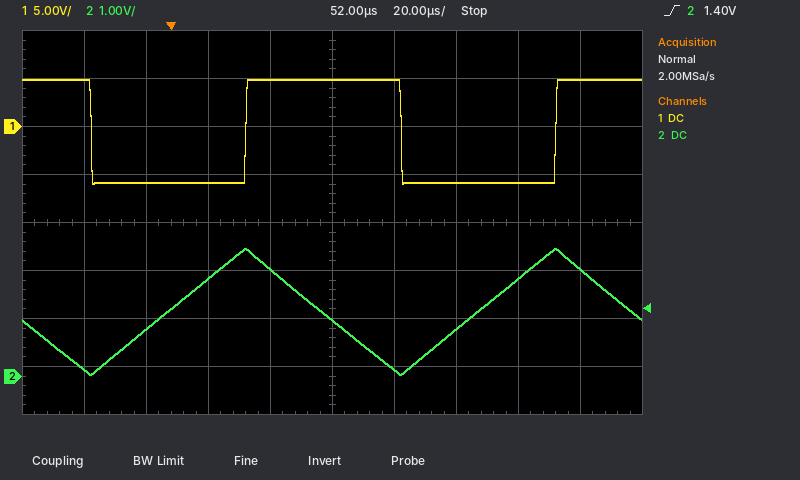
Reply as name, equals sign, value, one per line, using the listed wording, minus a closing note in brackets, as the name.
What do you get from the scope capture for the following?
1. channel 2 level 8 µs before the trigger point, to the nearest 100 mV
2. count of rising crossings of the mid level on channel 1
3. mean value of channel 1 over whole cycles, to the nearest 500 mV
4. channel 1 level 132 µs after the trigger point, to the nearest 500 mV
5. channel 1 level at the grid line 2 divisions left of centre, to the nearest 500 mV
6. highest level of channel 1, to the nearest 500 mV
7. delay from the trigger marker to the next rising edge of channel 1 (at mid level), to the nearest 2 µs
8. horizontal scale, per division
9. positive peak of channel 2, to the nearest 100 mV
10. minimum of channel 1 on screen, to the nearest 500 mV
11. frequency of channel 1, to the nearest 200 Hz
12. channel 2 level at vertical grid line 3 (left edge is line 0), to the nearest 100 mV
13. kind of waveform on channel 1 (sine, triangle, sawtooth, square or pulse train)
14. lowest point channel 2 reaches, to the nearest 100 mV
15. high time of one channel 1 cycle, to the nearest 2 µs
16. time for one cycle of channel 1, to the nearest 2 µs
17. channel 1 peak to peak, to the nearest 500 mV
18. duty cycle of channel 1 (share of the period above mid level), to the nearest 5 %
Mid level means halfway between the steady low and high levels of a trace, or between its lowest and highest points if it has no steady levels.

channel 2 level 8 µs before the trigger point, to the nearest 100 mV = 1.0 V
count of rising crossings of the mid level on channel 1 = 2
mean value of channel 1 over whole cycles, to the nearest 500 mV = -500 mV
channel 1 level 132 µs after the trigger point, to the nearest 500 mV = 5.0 V
channel 1 level at the grid line 2 divisions left of centre, to the nearest 500 mV = -6.0 V
highest level of channel 1, to the nearest 500 mV = 5.0 V
delay from the trigger marker to the next rising edge of channel 1 (at mid level), to the nearest 2 µs = 24 µs
horizontal scale, per division = 20 µs
positive peak of channel 2, to the nearest 100 mV = 2.7 V
minimum of channel 1 on screen, to the nearest 500 mV = -6.0 V
frequency of channel 1, to the nearest 200 Hz = 10.0 kHz
channel 2 level at vertical grid line 3 (left edge is line 0), to the nearest 100 mV = 2.0 V
kind of waveform on channel 1 = square
lowest point channel 2 reaches, to the nearest 100 mV = 0.0 V
high time of one channel 1 cycle, to the nearest 2 µs = 50 µs
time for one cycle of channel 1, to the nearest 2 µs = 100 µs
channel 1 peak to peak, to the nearest 500 mV = 11.0 V
duty cycle of channel 1 (share of the period above mid level), to the nearest 5 % = 50 %
